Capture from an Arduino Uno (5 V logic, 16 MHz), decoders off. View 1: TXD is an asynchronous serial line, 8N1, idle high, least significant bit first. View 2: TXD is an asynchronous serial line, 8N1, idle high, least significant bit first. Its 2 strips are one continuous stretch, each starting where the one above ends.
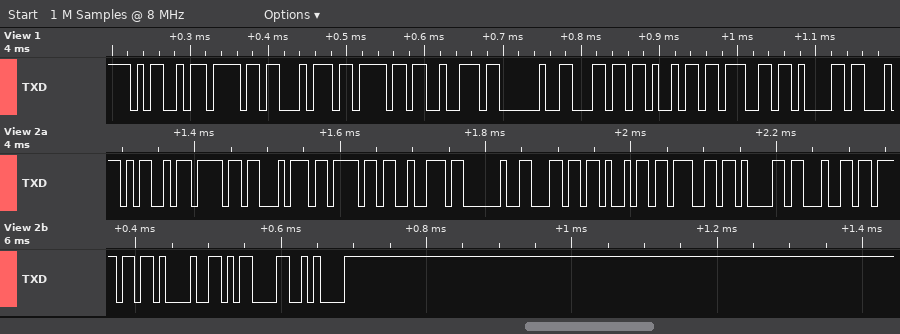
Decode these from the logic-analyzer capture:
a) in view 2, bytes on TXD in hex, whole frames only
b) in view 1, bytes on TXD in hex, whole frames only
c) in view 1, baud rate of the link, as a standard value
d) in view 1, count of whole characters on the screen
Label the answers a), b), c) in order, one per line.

a) 0x4D 0x6F 0x74 0x6F 0x72 0x20 0x6C 0x69 0x67 0x61 0x64 0x6F 0x21 0x0D 0x0A
b) 4D 6F 74 6F 72 20 6C 69 67 61
c) 115200 baud
d) 10
